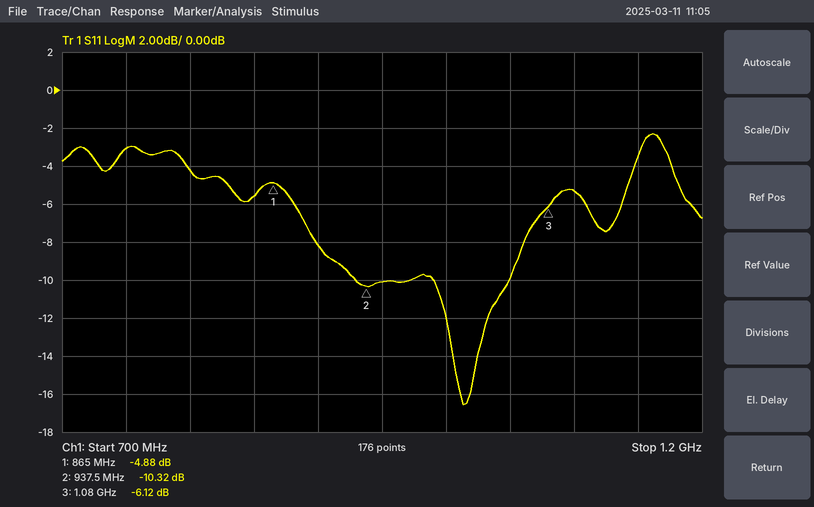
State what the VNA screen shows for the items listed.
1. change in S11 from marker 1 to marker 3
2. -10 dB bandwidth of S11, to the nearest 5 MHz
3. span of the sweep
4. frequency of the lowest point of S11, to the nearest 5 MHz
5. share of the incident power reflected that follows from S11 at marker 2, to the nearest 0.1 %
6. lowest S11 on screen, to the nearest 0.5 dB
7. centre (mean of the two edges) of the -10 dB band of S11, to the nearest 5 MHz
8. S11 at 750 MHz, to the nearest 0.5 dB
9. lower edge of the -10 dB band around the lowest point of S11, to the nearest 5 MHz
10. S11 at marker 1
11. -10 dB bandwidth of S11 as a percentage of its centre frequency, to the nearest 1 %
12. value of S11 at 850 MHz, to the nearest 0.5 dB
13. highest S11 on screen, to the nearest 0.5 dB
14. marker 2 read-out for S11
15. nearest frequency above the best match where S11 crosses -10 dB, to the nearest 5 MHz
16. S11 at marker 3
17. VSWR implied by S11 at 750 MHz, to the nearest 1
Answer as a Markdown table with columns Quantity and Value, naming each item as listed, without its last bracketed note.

| Quantity | Value |
|---|---|
| change in S11 from marker 1 to marker 3 | -1.24 dB |
| -10 dB bandwidth of S11, to the nearest 5 MHz | 60 MHz |
| span of the sweep | 500 MHz |
| frequency of the lowest point of S11, to the nearest 5 MHz | 1.015 GHz |
| share of the incident power reflected that follows from S11 at marker 2, to the nearest 0.1 % | 9.3 % |
| lowest S11 on screen, to the nearest 0.5 dB | -16.5 dB |
| centre (mean of the two edges) of the -10 dB band of S11, to the nearest 5 MHz | 1.020 GHz |
| S11 at 750 MHz, to the nearest 0.5 dB | -3.0 dB |
| lower edge of the -10 dB band around the lowest point of S11, to the nearest 5 MHz | 990 MHz |
| S11 at marker 1 | -4.88 dB |
| -10 dB bandwidth of S11 as a percentage of its centre frequency, to the nearest 1 % | 6 % |
| value of S11 at 850 MHz, to the nearest 0.5 dB | -5.5 dB |
| highest S11 on screen, to the nearest 0.5 dB | -2.5 dB |
| marker 2 read-out for S11 | -10.32 dB |
| nearest frequency above the best match where S11 crosses -10 dB, to the nearest 5 MHz | 1.050 GHz |
| S11 at marker 3 | -6.12 dB |
| VSWR implied by S11 at 750 MHz, to the nearest 1 | 6 |
